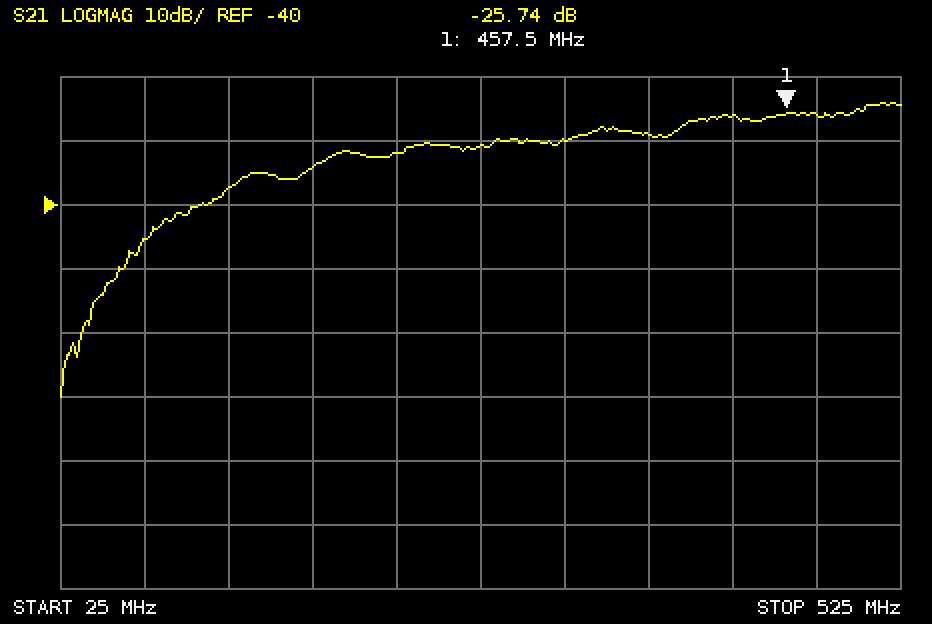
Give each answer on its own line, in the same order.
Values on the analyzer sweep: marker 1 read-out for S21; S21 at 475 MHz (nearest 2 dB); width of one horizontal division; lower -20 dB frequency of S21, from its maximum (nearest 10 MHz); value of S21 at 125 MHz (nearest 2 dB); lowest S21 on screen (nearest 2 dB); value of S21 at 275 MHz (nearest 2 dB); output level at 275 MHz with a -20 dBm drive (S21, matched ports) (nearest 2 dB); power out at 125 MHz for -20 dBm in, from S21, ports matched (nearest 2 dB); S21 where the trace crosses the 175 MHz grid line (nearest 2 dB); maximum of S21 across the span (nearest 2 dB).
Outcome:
-25.74 dB
-26 dB
50 MHz
80 MHz
-38 dB
-70 dB
-30 dB
-50 dBm
-58 dBm
-34 dB
-24 dB
